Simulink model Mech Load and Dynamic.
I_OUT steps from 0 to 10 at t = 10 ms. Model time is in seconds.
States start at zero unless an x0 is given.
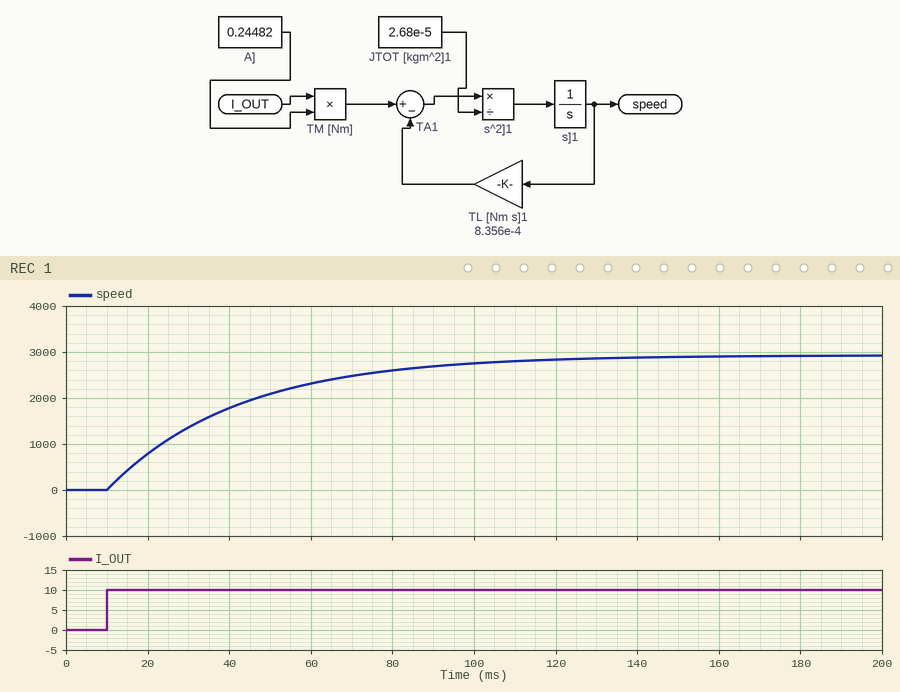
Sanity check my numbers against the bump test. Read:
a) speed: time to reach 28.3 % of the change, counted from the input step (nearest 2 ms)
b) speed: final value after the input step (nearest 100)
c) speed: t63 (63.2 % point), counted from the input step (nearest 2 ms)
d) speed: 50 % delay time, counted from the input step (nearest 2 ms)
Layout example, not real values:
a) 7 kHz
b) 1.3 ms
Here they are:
a) 10 ms
b) 2900
c) 32 ms
d) 22 ms
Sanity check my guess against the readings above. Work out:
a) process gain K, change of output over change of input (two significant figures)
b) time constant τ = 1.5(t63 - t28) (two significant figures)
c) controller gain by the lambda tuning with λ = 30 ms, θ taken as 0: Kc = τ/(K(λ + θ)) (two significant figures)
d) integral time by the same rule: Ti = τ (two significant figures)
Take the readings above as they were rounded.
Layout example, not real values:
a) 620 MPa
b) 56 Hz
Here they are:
a) 290
b) 33 ms
c) 0.0038
d) 33 ms
